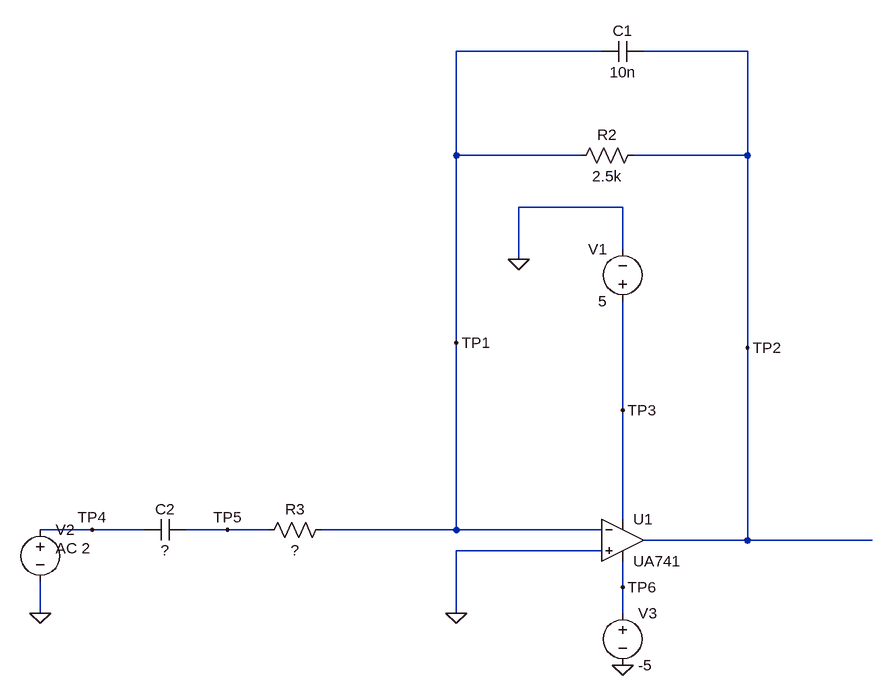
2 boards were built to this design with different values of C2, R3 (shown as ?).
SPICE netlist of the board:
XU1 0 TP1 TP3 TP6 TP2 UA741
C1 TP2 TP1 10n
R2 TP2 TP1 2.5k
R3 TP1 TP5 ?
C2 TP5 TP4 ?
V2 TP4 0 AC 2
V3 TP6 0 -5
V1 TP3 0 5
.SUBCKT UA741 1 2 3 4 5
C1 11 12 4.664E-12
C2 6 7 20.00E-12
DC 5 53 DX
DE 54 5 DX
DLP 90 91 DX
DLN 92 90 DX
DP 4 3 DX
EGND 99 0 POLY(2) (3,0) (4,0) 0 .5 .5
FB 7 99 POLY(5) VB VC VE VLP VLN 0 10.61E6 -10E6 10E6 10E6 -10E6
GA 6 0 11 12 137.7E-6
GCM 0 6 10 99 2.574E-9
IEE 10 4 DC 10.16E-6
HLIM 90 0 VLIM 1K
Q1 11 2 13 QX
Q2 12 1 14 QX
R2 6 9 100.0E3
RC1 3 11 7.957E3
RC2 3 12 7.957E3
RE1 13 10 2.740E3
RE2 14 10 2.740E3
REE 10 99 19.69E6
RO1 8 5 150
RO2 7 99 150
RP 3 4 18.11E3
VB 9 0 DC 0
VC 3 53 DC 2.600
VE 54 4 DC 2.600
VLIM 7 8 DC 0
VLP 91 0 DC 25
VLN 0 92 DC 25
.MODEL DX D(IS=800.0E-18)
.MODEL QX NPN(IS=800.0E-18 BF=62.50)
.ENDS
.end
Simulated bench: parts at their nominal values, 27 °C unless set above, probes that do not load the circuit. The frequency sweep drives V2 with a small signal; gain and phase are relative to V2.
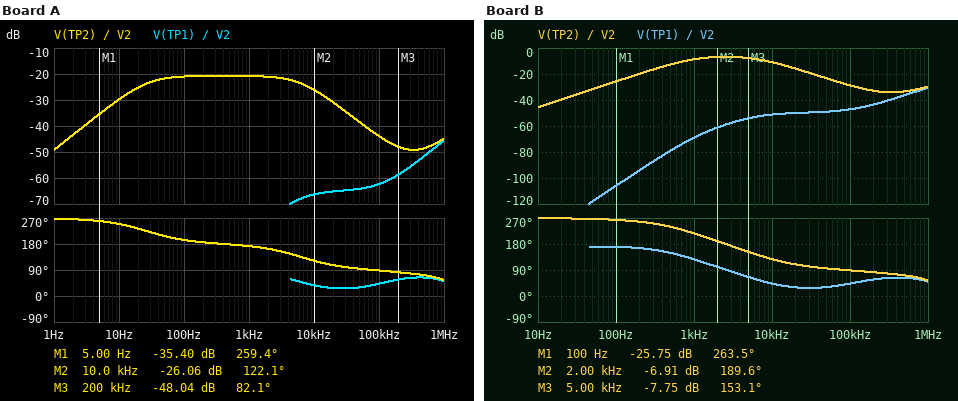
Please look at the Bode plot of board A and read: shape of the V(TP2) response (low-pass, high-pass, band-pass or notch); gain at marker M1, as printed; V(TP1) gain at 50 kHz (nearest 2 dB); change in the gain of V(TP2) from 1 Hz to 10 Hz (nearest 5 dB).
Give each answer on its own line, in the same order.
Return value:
band-pass
-35.40 dB
-64 dB
20 dB
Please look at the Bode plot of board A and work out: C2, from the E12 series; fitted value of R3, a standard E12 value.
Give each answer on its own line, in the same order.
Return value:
220 nF
27 kΩ
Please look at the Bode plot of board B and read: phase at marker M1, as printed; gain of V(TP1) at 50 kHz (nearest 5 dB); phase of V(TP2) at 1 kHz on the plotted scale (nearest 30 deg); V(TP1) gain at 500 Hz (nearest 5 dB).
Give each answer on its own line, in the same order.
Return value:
263.5 deg
-50 dB
210 deg
-80 dB
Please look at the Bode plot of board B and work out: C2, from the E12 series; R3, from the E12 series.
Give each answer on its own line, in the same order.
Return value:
33 nF
4.7 kΩ
